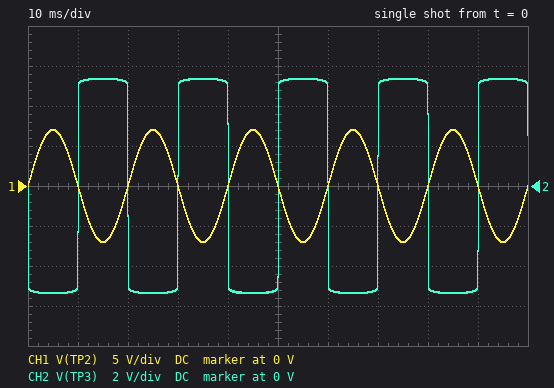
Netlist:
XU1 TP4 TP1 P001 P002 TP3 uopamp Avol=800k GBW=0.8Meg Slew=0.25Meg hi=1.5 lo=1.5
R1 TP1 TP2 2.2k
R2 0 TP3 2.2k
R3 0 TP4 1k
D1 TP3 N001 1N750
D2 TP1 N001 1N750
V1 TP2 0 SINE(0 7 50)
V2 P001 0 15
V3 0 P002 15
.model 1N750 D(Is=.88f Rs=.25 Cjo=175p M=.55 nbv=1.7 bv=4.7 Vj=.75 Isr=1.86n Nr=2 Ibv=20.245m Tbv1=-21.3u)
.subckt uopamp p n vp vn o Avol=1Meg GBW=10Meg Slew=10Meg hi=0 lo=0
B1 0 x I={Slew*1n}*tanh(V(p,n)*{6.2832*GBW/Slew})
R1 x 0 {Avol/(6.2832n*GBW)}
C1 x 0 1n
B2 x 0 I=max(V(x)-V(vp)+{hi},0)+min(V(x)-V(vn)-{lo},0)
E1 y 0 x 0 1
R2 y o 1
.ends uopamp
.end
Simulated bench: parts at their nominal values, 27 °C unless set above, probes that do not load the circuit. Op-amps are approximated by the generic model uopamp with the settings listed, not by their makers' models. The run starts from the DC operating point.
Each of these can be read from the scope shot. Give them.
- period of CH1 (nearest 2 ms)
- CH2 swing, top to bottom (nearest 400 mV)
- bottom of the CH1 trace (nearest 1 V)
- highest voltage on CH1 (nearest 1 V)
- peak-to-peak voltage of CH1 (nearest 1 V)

20 ms
10.8 V
-7 V
7 V
14 V
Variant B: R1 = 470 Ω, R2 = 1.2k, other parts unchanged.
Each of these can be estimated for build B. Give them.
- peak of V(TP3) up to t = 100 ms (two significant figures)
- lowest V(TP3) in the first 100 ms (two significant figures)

5.5 V
-5.5 V
